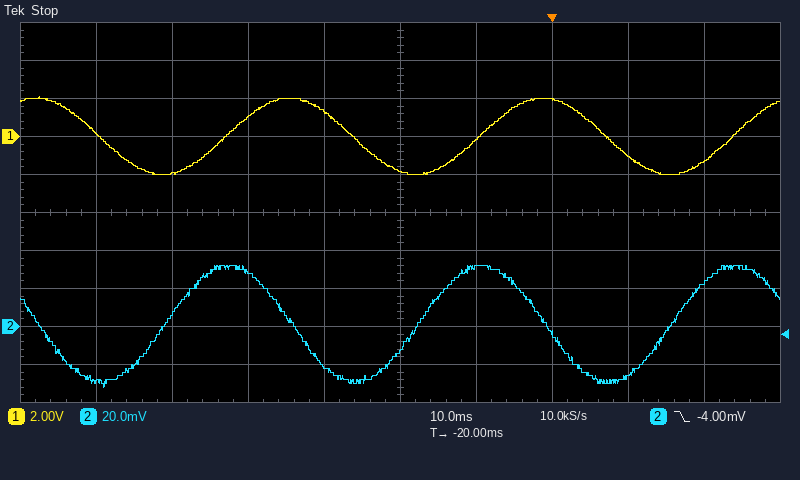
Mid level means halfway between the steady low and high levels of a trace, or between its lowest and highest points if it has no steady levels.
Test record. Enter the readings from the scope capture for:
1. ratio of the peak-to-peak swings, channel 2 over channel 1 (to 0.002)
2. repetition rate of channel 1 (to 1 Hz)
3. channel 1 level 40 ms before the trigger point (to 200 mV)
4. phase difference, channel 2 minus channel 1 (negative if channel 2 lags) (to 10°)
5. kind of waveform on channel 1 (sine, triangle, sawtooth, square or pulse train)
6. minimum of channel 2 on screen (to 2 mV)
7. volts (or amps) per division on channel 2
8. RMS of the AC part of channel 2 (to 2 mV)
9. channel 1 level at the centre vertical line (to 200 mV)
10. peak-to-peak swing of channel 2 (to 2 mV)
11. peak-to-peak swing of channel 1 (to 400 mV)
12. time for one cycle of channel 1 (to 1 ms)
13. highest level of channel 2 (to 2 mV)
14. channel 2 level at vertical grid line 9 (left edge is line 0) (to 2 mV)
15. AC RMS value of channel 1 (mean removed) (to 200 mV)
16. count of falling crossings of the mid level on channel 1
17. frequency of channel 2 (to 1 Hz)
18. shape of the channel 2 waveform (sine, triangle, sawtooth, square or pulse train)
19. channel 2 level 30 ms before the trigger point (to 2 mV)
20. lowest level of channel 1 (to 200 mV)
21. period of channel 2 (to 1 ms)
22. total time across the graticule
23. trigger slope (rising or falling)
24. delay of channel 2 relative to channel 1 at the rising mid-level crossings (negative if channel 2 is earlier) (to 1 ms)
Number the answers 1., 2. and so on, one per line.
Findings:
1. 0.016
2. 30 Hz
3. 1.0 V
4. +90°
5. sine
6. -32 mV
7. 20 mV
8. 22 mV
9. -1.8 V
10. 64 mV
11. 4.0 V
12. 33 ms
13. 32 mV
14. 24 mV
15. 1.4 V
16. 3
17. 30 Hz
18. sine
19. -20 mV
20. -2.0 V
21. 33 ms
22. 100 ms
23. falling
24. -8 ms
